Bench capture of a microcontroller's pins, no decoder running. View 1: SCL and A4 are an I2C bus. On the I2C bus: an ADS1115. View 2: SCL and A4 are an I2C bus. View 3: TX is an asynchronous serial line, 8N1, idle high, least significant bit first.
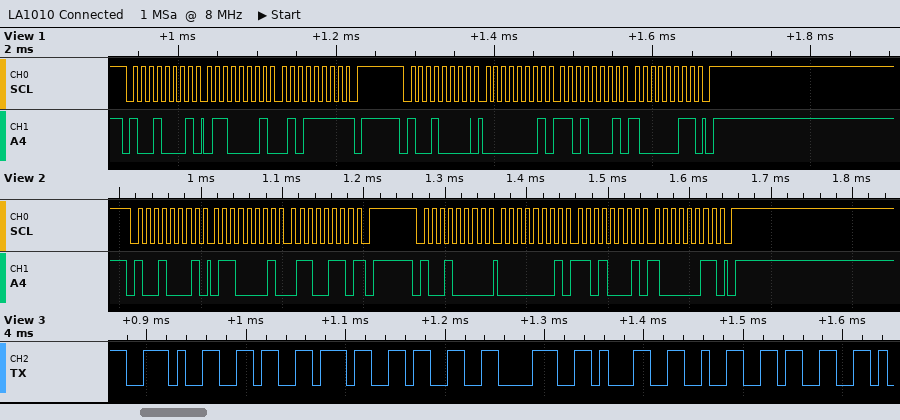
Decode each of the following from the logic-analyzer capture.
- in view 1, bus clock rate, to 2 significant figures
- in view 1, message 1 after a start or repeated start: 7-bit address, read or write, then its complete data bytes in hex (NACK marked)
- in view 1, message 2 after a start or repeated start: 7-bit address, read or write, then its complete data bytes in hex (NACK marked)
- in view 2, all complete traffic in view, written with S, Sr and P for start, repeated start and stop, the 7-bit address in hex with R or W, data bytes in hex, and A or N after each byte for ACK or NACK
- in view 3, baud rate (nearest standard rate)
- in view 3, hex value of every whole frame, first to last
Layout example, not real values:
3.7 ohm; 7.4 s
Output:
100 kHz; 0x48 read: 61 5F NACK; 0x48 write: 01 D1 83; S 48R A 61 A 66 N P S 48W A 01 A D1 A 83 A P; 115200 baud; 0x2E 0x36 0x37 0x33 0x38 0x31 0x32 0x33
